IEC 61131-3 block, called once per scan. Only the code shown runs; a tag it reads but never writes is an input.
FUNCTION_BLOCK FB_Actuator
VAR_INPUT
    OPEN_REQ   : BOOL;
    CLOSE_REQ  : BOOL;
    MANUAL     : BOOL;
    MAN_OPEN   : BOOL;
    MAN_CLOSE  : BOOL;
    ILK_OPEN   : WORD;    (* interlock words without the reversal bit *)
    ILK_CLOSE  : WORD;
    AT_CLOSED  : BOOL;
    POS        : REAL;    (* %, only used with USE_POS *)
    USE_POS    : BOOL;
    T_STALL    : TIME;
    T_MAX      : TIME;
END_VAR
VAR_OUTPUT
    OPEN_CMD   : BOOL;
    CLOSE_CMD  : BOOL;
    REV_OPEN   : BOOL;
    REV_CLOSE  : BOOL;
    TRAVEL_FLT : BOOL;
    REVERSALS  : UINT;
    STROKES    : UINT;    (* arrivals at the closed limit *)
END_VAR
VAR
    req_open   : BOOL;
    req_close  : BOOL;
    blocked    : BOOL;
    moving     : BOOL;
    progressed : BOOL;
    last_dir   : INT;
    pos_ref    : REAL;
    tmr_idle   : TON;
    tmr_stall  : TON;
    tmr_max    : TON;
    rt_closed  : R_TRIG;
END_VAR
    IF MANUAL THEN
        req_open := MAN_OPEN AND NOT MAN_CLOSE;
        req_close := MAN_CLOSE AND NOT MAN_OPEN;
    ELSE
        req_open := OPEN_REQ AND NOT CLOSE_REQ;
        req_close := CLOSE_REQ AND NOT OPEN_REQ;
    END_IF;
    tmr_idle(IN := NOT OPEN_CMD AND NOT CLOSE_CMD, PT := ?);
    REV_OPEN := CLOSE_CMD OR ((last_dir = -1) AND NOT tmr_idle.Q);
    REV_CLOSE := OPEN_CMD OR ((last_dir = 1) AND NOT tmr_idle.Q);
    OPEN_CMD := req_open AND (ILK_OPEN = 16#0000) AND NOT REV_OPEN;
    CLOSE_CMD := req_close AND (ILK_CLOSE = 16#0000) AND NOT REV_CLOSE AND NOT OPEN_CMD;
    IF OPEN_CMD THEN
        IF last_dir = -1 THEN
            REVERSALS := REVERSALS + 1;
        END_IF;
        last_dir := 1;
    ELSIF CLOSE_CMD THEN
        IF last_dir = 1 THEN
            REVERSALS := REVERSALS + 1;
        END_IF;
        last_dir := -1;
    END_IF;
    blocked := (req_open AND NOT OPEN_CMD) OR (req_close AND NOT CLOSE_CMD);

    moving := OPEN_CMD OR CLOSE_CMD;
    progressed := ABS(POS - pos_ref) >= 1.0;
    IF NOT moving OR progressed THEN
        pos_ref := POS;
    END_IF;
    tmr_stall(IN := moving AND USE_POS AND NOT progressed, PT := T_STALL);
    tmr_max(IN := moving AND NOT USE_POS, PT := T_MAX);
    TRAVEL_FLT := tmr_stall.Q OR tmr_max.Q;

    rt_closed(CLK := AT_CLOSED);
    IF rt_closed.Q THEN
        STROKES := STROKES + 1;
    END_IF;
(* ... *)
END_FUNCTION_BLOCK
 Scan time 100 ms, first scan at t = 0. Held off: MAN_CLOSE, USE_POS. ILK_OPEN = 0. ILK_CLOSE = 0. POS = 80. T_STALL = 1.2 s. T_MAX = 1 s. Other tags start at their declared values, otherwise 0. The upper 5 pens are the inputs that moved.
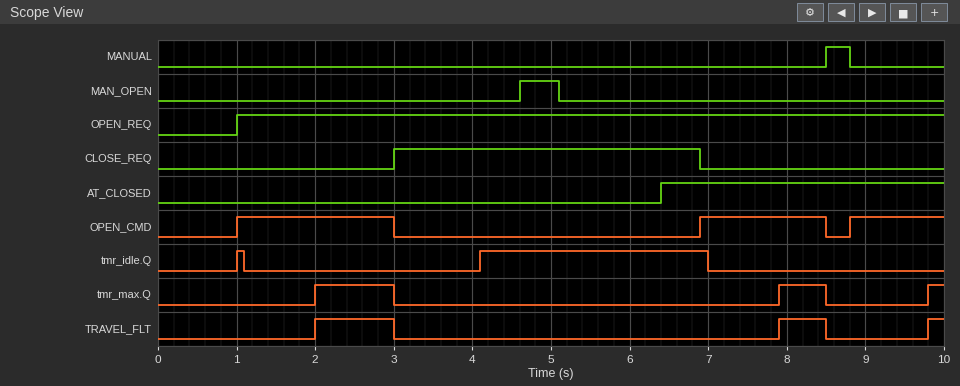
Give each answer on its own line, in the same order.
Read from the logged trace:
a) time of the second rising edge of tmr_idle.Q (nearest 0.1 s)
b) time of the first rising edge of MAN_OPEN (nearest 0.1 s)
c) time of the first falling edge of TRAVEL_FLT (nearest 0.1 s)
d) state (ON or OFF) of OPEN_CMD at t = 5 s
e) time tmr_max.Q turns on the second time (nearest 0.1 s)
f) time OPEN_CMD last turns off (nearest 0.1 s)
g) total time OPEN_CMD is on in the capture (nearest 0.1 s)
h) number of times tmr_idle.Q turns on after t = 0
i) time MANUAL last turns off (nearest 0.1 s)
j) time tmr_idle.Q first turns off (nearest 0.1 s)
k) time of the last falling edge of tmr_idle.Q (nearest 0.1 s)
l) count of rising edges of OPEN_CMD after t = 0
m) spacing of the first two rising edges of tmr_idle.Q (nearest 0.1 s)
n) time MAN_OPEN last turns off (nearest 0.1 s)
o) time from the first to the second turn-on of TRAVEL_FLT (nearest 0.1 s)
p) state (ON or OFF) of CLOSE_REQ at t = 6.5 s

4.1 s
4.6 s
3.0 s
OFF
7.9 s
8.5 s
4.8 s
2
8.8 s
1.1 s
7.0 s
3
3.1 s
5.1 s
5.9 s
ON
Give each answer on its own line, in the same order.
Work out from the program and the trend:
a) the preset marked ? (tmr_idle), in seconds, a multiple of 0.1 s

1.0 s
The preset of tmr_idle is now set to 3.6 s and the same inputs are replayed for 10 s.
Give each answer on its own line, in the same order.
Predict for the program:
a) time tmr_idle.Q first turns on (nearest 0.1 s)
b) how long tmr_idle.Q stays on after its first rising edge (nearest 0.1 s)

6.7 s
0.3 s
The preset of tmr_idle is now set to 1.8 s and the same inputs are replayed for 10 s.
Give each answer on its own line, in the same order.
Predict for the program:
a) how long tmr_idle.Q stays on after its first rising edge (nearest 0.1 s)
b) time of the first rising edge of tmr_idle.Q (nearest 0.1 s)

2.1 s
4.9 s
